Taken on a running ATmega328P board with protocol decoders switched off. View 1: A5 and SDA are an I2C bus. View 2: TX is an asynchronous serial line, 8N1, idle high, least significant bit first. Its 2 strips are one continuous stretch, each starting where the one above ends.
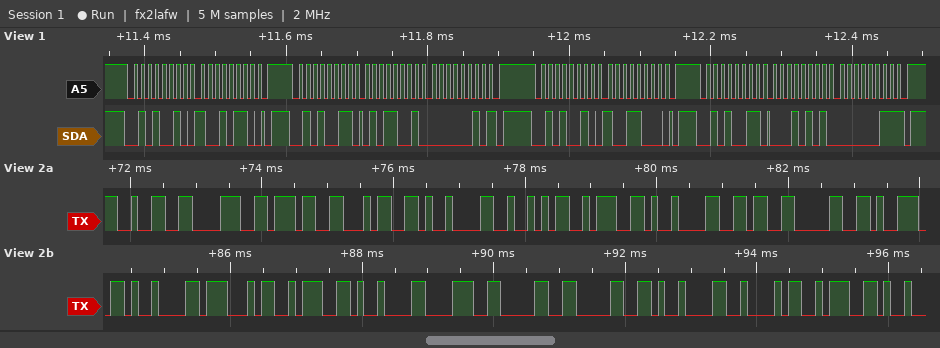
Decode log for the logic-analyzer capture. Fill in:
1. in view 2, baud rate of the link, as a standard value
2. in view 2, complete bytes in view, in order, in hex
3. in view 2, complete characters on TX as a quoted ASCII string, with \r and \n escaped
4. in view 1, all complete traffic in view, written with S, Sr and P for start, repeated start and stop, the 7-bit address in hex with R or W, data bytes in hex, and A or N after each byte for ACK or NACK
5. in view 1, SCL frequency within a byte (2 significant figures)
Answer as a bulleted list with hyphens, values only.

- 9600 baud
- 32 38 37 34 09 52 3A 09 36 30 39 09 47 3A 09 38 30 30 09 42 3A
- "2874\tR:\t609\tG:\t800\tB:"
- S 29W A 96 A P S 29R A 59 A 02 N P S 29W A 98 A P S 29R A 15 A 03 N P
- 100 kHz
